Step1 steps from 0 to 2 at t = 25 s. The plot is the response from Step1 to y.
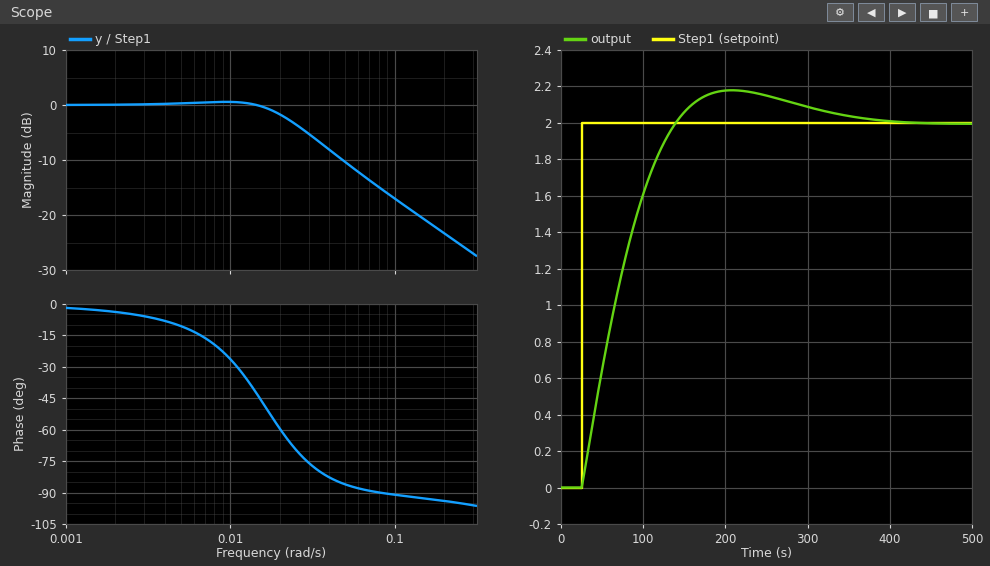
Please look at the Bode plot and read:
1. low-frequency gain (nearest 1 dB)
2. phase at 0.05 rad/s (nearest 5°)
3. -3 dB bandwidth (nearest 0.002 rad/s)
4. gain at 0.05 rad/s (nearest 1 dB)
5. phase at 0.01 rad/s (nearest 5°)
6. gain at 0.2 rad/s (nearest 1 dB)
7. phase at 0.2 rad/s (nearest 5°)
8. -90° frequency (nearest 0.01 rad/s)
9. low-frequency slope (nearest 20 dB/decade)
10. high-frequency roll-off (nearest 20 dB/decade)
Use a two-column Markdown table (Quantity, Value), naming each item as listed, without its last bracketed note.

| Quantity | Value |
|---|---|
| low-frequency gain | 0 dB |
| phase at 0.05 rad/s | -85° |
| -3 dB bandwidth | 0.024 rad/s |
| gain at 0.05 rad/s | -10 dB |
| phase at 0.01 rad/s | -25° |
| gain at 0.2 rad/s | -23 dB |
| phase at 0.2 rad/s | -95° |
| -90° frequency | 0.08 rad/s |
| low-frequency slope | 0 dB/decade |
| high-frequency roll-off | -20 dB/decade |
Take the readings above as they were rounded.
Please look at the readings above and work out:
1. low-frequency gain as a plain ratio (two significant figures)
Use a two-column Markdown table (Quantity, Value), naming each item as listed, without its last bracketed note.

| Quantity | Value |
|---|---|
| low-frequency gain as a plain ratio | 1.0 |
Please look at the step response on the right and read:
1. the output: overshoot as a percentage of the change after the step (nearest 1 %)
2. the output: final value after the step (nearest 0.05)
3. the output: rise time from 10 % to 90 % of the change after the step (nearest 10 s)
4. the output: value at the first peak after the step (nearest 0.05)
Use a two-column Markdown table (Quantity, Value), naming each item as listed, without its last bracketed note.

| Quantity | Value |
|---|---|
| the output: overshoot as a percentage of the change after the step | 9 % |
| the output: final value after the step | 2.00 |
| the output: rise time from 10 % to 90 % of the change after the step | 80 s |
| the output: value at the first peak after the step | 2.20 |
